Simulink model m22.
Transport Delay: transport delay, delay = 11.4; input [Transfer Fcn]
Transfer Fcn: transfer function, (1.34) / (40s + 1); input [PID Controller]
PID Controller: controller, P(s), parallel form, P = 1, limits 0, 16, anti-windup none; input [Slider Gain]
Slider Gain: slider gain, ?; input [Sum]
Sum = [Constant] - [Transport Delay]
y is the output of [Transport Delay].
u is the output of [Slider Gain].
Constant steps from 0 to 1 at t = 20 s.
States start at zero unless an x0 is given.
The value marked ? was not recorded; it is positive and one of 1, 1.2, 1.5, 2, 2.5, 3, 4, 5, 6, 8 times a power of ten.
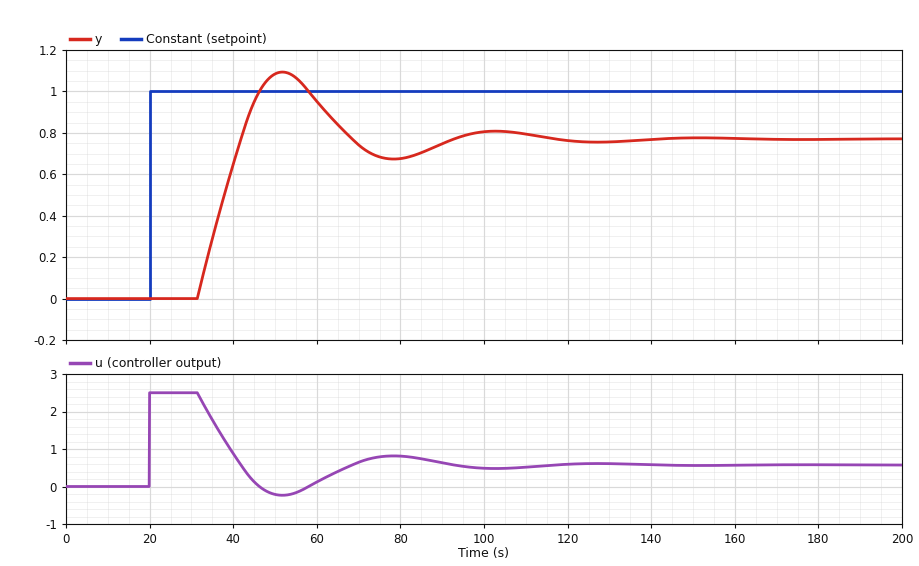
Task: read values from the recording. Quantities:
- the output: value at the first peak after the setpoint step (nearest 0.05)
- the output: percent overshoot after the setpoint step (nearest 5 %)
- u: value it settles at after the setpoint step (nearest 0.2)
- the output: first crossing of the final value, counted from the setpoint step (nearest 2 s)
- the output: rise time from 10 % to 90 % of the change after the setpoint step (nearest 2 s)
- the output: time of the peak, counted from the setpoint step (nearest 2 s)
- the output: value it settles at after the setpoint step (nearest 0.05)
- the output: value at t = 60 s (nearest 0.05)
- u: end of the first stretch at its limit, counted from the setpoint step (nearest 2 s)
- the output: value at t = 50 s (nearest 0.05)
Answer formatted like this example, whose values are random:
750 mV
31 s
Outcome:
1.10
40 %
0.6
22 s
8 s
32 s
0.75
0.95
12 s
1.10
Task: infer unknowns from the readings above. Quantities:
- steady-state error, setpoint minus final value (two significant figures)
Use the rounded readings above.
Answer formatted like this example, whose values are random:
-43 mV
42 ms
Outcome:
0.25
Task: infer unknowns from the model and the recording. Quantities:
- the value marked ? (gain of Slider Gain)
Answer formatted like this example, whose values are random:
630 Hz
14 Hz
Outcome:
2.5
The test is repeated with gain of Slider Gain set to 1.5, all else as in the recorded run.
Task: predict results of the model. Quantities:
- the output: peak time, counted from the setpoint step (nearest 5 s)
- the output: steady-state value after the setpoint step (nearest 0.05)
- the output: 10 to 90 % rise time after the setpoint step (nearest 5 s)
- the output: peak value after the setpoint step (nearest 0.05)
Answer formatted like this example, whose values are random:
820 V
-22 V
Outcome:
40 s
0.65
15 s
0.75
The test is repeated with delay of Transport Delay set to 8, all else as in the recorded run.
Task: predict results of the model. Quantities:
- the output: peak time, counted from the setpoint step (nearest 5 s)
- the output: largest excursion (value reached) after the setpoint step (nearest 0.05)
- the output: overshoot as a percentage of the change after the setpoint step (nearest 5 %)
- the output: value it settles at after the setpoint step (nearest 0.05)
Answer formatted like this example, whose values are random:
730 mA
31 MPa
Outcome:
25 s
0.90
20 %
0.75
